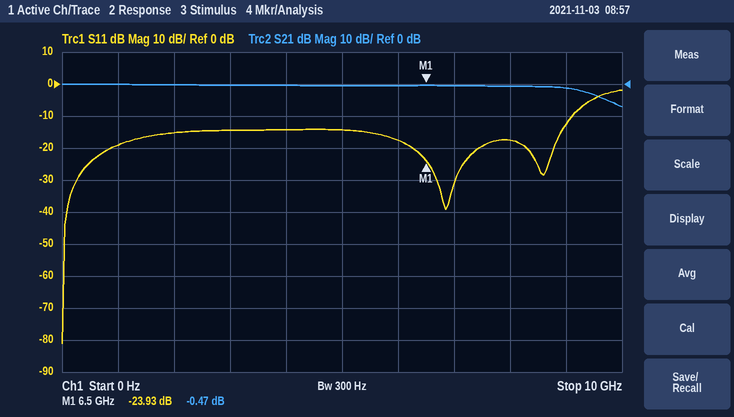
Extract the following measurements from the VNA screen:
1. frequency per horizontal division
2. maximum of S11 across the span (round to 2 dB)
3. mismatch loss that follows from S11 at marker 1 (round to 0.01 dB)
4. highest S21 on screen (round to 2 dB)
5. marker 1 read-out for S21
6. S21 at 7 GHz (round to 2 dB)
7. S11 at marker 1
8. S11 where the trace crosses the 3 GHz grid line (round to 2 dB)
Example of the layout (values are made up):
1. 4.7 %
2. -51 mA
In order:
1. 1 GHz
2. -2 dB
3. 0.02 dB
4. 0 dB
5. -0.47 dB
6. 0 dB
7. -23.93 dB
8. -14 dB
